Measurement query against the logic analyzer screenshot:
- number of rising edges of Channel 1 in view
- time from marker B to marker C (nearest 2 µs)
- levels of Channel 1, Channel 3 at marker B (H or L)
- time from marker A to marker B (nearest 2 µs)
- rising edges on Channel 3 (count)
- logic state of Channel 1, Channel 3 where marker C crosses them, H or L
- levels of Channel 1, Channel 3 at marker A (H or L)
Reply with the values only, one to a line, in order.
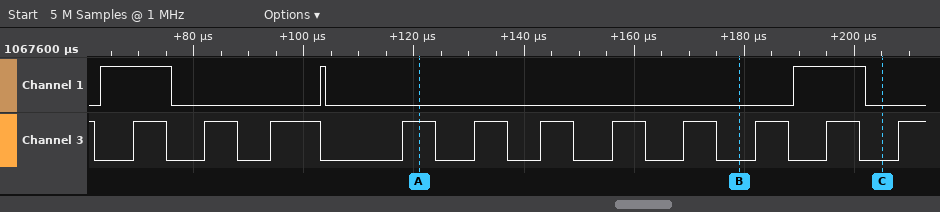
3
26 µs
Channel 1=L, Channel 3=L
58 µs
11
Channel 1=L, Channel 3=L
Channel 1=L, Channel 3=H
